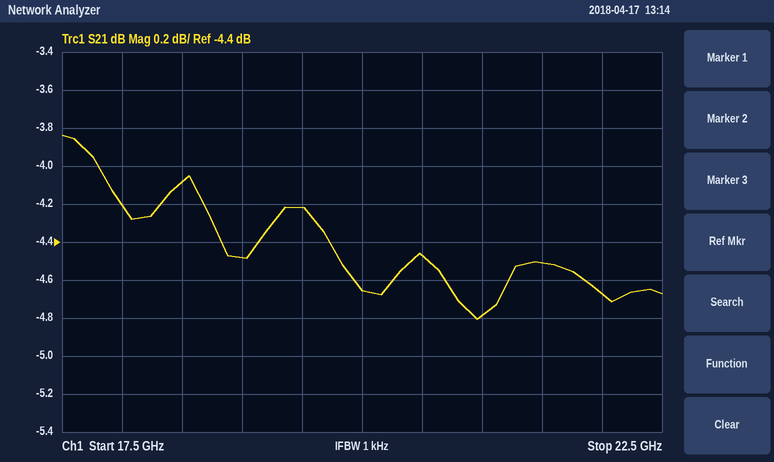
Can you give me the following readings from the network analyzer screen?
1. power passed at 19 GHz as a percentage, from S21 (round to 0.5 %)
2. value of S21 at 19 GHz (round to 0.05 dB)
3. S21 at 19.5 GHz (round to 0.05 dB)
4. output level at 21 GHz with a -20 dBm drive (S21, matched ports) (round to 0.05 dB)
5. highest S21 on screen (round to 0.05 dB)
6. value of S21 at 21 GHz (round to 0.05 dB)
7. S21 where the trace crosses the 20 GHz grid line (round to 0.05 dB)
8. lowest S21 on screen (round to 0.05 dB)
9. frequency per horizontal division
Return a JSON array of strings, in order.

["35.5 %", "-4.50 dB", "-4.20 dB", "-24.80 dBm", "-3.85 dB", "-4.80 dB", "-4.65 dB", "-4.80 dB", "500 MHz"]
